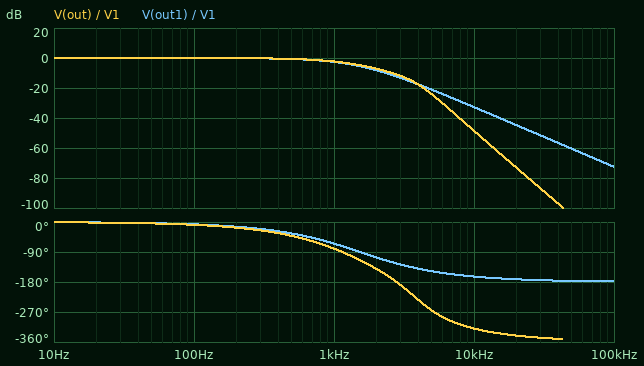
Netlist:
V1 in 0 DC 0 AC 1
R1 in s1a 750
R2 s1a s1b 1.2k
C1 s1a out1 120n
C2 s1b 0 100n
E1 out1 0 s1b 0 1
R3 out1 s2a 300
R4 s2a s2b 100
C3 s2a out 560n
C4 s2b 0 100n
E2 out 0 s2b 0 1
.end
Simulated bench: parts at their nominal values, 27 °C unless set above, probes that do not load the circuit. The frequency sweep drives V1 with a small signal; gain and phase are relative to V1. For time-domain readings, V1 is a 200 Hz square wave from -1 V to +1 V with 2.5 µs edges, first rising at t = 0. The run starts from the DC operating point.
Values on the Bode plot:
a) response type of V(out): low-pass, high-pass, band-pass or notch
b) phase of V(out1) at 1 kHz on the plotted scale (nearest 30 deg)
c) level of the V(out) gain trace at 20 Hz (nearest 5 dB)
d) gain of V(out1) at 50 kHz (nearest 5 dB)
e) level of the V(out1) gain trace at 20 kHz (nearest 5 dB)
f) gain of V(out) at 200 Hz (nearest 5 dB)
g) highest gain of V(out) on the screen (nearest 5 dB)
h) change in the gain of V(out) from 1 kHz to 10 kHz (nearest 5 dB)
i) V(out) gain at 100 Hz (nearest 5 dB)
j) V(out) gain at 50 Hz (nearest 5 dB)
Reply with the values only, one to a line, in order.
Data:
low-pass
-60 deg
0 dB
-60 dB
-45 dB
0 dB
0 dB
-45 dB
0 dB
0 dB
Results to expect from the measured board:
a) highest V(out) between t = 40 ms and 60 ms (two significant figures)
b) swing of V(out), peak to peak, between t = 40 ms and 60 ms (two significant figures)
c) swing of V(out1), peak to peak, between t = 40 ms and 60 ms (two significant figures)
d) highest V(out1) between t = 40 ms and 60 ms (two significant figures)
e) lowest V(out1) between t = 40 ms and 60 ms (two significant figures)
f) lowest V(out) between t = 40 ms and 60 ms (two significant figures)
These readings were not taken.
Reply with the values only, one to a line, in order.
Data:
1.0 V
2.0 V
2.0 V
1.0 V
-1.0 V
-1.0 V
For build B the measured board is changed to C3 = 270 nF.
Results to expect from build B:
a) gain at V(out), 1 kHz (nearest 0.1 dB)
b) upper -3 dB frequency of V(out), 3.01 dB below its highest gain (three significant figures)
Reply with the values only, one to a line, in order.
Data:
-2.6 dB
1.08 kHz
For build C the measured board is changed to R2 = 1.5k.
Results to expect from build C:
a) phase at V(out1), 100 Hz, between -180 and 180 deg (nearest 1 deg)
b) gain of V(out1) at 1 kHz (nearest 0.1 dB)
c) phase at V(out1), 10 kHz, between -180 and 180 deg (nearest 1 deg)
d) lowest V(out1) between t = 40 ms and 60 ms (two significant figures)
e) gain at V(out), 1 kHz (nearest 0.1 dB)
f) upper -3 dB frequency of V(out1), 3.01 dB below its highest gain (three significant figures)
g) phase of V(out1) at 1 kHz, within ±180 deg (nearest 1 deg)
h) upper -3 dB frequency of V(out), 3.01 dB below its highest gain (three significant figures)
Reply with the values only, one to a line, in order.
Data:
-8 deg
-3.5 dB
-165 deg
-1.0 V
-3.2 dB
923 Hz
-72 deg
971 Hz
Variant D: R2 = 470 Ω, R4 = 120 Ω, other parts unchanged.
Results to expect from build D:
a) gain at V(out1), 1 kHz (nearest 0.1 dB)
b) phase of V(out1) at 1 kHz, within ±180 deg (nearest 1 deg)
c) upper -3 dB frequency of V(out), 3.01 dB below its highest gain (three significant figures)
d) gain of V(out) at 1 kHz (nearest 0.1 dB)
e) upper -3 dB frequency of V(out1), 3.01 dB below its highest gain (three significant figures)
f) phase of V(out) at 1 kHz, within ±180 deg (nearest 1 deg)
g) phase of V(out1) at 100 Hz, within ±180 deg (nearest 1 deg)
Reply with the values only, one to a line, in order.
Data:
-1.1 dB
-43 deg
2.15 kHz
-0.7 dB
1.72 kHz
-59 deg
-4 deg
